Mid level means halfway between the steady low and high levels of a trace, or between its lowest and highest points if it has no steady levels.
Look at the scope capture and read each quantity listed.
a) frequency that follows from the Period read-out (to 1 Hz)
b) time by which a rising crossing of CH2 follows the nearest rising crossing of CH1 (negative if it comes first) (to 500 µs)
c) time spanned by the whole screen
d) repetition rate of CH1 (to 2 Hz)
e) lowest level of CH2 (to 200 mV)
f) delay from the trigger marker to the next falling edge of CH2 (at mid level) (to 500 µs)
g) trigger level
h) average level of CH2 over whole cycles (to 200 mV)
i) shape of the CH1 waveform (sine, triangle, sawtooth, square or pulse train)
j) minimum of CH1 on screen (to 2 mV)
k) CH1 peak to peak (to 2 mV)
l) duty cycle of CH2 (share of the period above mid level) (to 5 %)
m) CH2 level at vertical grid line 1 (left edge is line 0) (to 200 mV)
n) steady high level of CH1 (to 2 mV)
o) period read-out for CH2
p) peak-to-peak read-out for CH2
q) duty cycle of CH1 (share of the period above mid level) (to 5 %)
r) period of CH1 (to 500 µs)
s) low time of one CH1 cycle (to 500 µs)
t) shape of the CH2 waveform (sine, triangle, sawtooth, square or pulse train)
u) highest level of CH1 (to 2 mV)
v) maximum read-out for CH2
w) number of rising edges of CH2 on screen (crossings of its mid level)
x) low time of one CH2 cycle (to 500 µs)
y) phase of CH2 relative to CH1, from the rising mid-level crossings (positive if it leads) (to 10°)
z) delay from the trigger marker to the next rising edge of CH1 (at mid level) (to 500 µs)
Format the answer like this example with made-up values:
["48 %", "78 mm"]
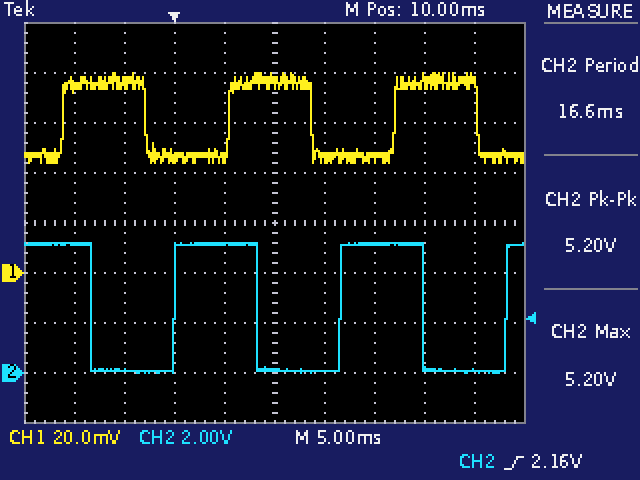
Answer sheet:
["60 Hz", "-5.5 ms", "50 ms", "60 Hz", "0.0 V", "8.5 ms", "2.16 V", "2.6 V", "square", "44 mV", "36 mV", "50 %", "5.2 V", "76 mV", "16.6 ms", "5.20 V", "50 %", "16.5 ms", "8.5 ms", "square", "80 mV", "5.20 V", "3", "8.5 ms", "+120°", "5.5 ms"]
